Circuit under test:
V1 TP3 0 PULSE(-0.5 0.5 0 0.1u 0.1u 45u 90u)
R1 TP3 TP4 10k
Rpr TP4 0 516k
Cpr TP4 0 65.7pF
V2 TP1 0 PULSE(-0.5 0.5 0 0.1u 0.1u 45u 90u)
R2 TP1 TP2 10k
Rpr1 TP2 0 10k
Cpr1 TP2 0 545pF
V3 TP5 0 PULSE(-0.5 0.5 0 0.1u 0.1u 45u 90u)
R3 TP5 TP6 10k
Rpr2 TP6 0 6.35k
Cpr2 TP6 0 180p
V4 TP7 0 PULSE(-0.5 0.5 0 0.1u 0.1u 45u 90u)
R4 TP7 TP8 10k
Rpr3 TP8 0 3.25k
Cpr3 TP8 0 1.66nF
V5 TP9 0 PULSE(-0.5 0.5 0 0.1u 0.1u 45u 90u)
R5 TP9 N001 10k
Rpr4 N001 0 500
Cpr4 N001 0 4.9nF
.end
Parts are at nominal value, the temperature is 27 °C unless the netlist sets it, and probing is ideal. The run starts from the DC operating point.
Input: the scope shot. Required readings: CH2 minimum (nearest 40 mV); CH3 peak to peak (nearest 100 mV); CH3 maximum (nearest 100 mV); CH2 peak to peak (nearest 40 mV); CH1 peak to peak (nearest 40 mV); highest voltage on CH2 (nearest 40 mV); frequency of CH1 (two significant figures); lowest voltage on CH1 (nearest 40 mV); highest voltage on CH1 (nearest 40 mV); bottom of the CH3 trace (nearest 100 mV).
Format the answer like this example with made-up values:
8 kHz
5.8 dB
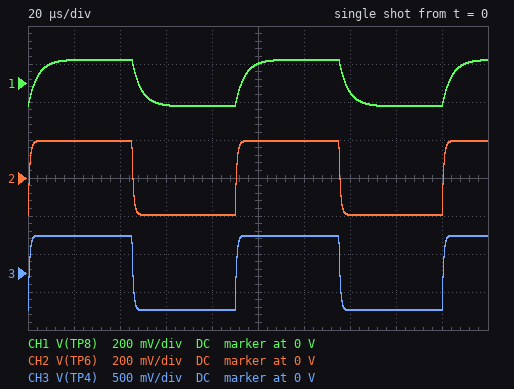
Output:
-200 mV
1.0 V
500 mV
400 mV
240 mV
200 mV
11 kHz
-120 mV
120 mV
-500 mV
